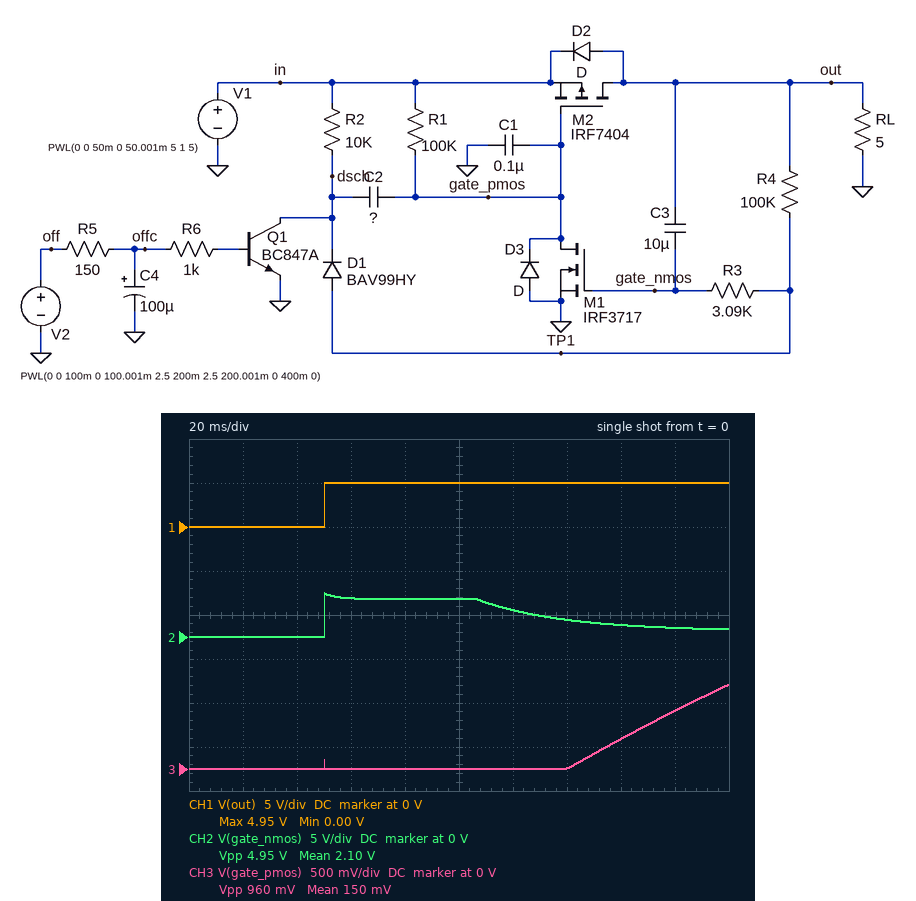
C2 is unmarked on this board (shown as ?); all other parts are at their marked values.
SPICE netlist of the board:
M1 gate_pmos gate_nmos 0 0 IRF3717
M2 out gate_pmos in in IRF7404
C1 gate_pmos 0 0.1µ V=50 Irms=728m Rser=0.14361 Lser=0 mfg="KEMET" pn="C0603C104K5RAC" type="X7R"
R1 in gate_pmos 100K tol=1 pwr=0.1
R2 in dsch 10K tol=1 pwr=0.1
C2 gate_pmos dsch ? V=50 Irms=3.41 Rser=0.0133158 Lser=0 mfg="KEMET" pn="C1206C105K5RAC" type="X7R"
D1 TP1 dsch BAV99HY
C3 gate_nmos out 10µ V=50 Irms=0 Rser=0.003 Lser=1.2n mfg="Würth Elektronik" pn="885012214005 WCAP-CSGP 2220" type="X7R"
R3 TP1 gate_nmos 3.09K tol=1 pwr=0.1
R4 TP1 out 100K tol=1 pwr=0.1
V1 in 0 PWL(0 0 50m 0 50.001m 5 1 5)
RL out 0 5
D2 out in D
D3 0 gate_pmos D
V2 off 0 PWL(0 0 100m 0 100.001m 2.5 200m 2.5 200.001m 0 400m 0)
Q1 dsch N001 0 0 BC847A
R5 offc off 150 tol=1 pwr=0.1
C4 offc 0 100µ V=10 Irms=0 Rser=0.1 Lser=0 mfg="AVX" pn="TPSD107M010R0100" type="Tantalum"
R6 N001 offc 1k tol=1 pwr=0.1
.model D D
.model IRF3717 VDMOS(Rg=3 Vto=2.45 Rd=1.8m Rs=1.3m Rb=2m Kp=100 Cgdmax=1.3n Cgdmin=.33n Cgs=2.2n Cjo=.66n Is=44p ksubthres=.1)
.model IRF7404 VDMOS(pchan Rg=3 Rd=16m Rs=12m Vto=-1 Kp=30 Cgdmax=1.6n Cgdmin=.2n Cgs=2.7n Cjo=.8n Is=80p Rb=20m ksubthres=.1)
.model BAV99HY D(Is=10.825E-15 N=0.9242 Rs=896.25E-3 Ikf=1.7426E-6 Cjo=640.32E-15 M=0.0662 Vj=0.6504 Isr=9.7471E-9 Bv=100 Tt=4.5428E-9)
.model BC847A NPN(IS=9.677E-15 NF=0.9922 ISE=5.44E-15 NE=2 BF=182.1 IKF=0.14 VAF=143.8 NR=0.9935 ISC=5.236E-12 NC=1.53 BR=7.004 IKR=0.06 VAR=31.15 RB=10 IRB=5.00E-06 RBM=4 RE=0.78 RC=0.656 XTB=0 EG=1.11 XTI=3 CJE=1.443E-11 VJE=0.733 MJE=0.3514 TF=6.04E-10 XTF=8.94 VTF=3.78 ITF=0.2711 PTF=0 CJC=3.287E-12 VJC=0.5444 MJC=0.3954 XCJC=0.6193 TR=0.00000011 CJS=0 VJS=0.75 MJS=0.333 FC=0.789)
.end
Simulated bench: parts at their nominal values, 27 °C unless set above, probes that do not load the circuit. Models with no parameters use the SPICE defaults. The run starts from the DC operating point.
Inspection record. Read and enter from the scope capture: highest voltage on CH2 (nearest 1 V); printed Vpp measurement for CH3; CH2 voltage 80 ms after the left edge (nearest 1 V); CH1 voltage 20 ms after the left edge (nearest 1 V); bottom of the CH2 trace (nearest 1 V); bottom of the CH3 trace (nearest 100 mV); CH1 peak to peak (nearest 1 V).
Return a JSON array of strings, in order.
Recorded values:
["5 V", "960 mV", "4 V", "0 V", "0 V", "0 V", "5 V"]
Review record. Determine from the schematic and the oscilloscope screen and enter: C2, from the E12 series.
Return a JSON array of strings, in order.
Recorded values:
["2.7 µF"]
